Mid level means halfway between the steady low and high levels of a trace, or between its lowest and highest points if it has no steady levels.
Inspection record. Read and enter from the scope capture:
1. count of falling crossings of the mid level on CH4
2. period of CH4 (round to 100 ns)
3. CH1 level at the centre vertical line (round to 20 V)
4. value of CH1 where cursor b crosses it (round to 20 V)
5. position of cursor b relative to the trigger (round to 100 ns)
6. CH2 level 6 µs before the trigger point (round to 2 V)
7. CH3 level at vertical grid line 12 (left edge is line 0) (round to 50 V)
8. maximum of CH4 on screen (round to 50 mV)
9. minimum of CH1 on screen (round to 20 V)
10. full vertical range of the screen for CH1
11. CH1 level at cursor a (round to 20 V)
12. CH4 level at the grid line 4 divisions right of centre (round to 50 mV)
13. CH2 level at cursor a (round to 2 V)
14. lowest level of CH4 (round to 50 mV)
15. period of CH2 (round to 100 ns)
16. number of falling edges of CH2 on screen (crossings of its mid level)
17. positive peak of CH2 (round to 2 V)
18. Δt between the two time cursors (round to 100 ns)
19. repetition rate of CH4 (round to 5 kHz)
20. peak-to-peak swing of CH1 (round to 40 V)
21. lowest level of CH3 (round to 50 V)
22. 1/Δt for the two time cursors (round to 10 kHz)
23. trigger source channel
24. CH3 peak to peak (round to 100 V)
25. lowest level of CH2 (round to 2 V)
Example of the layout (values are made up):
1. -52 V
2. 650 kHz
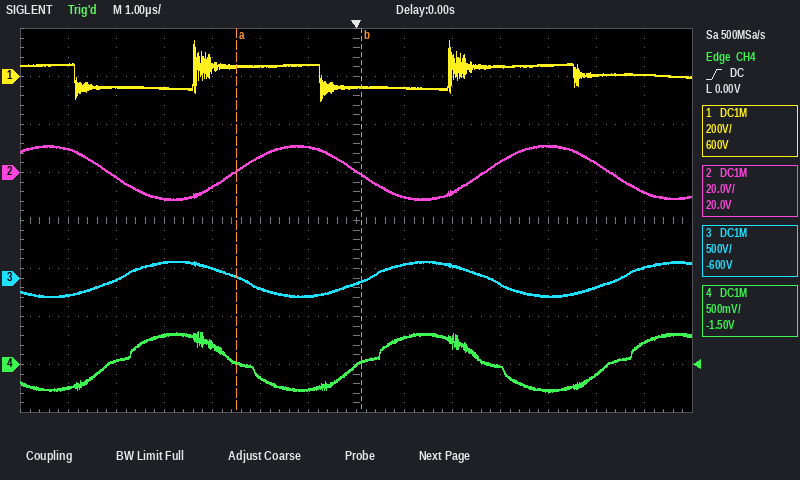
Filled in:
1. 2
2. 5.2 µs
3. -40 V
4. -40 V
5. +100 ns
6. 10 V
7. -100 V
8. 350 mV
9. -100 V
10. 1.6 kV
11. 40 V
12. -250 mV
13. 0 V
14. -300 mV
15. 5.2 µs
16. 3
17. 12 V
18. 2.6 µs
19. 190 kHz
20. 240 V
21. -200 V
22. 380 kHz
23. CH4
24. 400 V
25. -12 V
